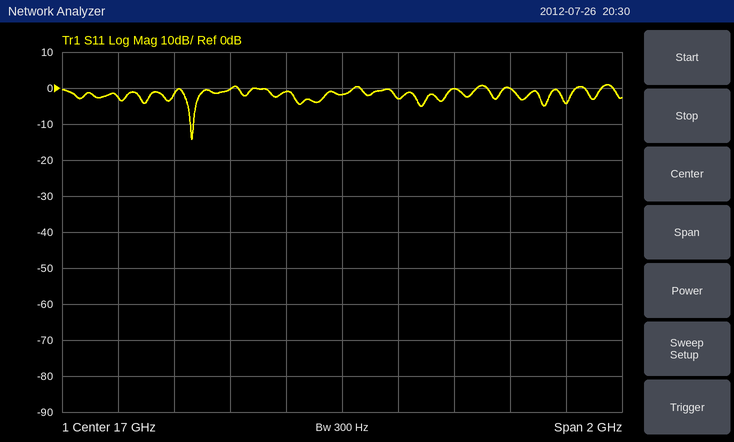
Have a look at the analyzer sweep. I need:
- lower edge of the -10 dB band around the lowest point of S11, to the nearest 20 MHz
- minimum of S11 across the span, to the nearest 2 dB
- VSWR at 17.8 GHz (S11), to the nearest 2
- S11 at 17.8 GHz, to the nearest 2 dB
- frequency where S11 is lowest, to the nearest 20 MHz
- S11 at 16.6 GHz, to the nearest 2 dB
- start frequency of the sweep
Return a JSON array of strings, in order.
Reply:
["16.46 GHz", "-14 dB", "4", "-4 dB", "16.46 GHz", "0 dB", "16 GHz"]
